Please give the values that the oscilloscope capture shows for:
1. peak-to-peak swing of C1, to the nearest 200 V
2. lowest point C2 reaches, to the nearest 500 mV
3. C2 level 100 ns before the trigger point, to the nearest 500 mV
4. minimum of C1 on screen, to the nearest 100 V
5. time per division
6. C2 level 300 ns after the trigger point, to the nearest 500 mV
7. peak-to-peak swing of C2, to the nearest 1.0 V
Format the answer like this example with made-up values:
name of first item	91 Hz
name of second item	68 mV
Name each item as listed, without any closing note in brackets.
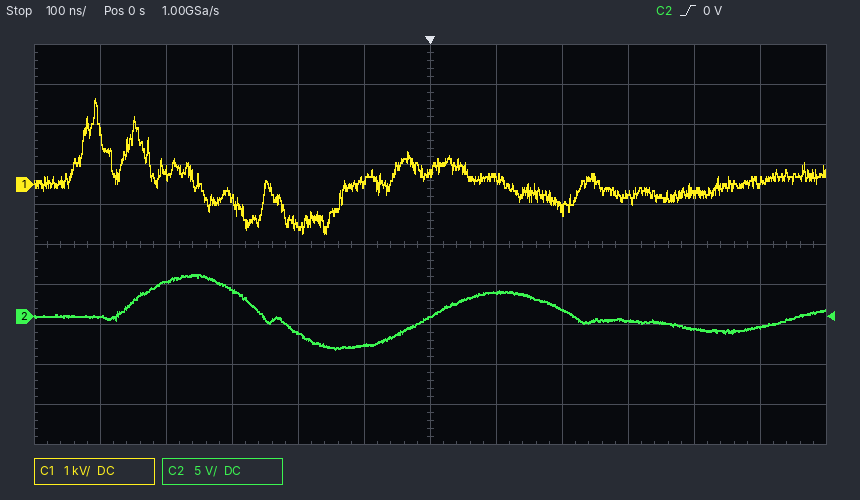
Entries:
peak-to-peak swing of C1, to the nearest 200 V	3.4 kV
lowest point C2 reaches, to the nearest 500 mV	-4.0 V
C2 level 100 ns before the trigger point, to the nearest 500 mV	-3.5 V
minimum of C1 on screen, to the nearest 100 V	-1.2 kV
time per division	100 ns
C2 level 300 ns after the trigger point, to the nearest 500 mV	-500 mV
peak-to-peak swing of C2, to the nearest 1.0 V	9.0 V
